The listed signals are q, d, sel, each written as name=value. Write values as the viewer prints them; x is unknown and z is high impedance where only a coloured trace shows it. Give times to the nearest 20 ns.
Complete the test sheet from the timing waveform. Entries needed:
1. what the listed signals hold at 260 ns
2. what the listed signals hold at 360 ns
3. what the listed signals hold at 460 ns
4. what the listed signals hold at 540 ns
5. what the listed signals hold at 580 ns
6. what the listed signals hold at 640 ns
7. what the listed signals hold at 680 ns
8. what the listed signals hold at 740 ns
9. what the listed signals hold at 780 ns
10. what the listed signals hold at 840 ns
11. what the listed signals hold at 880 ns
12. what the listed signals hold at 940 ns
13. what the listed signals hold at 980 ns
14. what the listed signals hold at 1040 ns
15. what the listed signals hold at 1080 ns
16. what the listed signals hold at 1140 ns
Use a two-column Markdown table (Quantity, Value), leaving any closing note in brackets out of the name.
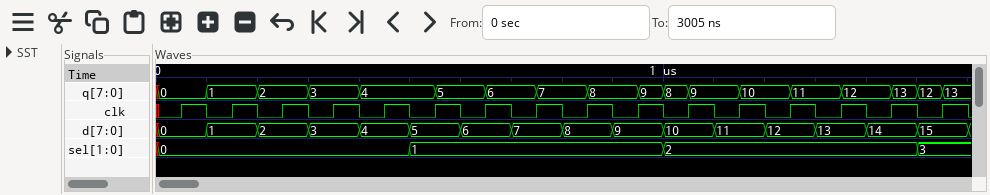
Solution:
| Quantity | Value |
|---|---|
| what the listed signals hold at 260 ns | q=2, d=2, sel=0 |
| what the listed signals hold at 360 ns | q=3, d=3, sel=0 |
| what the listed signals hold at 460 ns | q=4, d=4, sel=0 |
| what the listed signals hold at 540 ns | q=4, d=5, sel=1 |
| what the listed signals hold at 580 ns | q=5, d=5, sel=1 |
| what the listed signals hold at 640 ns | q=5, d=6, sel=1 |
| what the listed signals hold at 680 ns | q=6, d=6, sel=1 |
| what the listed signals hold at 740 ns | q=6, d=7, sel=1 |
| what the listed signals hold at 780 ns | q=7, d=7, sel=1 |
| what the listed signals hold at 840 ns | q=7, d=8, sel=1 |
| what the listed signals hold at 880 ns | q=8, d=8, sel=1 |
| what the listed signals hold at 940 ns | q=8, d=9, sel=1 |
| what the listed signals hold at 980 ns | q=9, d=9, sel=1 |
| what the listed signals hold at 1040 ns | q=8, d=10, sel=2 |
| what the listed signals hold at 1080 ns | q=9, d=10, sel=2 |
| what the listed signals hold at 1140 ns | q=9, d=11, sel=2 |
